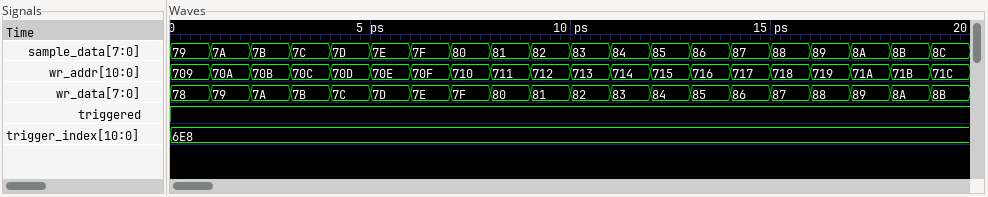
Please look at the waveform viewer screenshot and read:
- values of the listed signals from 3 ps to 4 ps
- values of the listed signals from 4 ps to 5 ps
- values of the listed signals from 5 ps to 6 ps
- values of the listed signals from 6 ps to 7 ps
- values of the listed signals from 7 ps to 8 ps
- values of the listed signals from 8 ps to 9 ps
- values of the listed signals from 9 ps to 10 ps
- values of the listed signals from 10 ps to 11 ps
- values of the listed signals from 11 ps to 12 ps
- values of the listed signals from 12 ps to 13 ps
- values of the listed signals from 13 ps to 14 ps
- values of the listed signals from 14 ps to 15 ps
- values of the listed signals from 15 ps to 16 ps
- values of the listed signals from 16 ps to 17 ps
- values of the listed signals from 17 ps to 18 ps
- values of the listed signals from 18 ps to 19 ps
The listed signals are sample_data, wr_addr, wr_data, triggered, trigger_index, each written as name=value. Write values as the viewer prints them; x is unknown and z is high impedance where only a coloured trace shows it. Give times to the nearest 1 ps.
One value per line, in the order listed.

sample_data=7C, wr_addr=70C, wr_data=7B, triggered=1, trigger_index=6E8
sample_data=7D, wr_addr=70D, wr_data=7C, triggered=1, trigger_index=6E8
sample_data=7E, wr_addr=70E, wr_data=7D, triggered=1, trigger_index=6E8
sample_data=7F, wr_addr=70F, wr_data=7E, triggered=1, trigger_index=6E8
sample_data=80, wr_addr=710, wr_data=7F, triggered=1, trigger_index=6E8
sample_data=81, wr_addr=711, wr_data=80, triggered=1, trigger_index=6E8
sample_data=82, wr_addr=712, wr_data=81, triggered=1, trigger_index=6E8
sample_data=83, wr_addr=713, wr_data=82, triggered=1, trigger_index=6E8
sample_data=84, wr_addr=714, wr_data=83, triggered=1, trigger_index=6E8
sample_data=85, wr_addr=715, wr_data=84, triggered=1, trigger_index=6E8
sample_data=86, wr_addr=716, wr_data=85, triggered=1, trigger_index=6E8
sample_data=87, wr_addr=717, wr_data=86, triggered=1, trigger_index=6E8
sample_data=88, wr_addr=718, wr_data=87, triggered=1, trigger_index=6E8
sample_data=89, wr_addr=719, wr_data=88, triggered=1, trigger_index=6E8
sample_data=8A, wr_addr=71A, wr_data=89, triggered=1, trigger_index=6E8
sample_data=8B, wr_addr=71B, wr_data=8A, triggered=1, trigger_index=6E8
